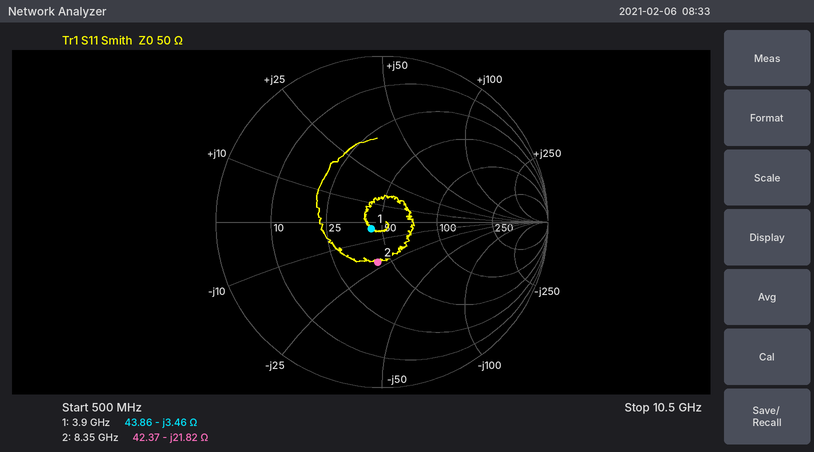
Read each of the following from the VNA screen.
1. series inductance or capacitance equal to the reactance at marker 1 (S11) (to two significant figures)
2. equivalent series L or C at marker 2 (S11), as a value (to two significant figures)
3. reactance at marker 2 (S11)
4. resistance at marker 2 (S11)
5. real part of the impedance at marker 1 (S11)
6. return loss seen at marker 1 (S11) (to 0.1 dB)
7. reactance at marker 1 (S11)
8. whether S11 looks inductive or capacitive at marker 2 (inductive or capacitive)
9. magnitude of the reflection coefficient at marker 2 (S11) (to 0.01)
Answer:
12 pF
870 fF
-21.82 Ω
42.37 Ω
43.86 Ω
22.5 dB
-3.46 Ω
capacitive
0.24
